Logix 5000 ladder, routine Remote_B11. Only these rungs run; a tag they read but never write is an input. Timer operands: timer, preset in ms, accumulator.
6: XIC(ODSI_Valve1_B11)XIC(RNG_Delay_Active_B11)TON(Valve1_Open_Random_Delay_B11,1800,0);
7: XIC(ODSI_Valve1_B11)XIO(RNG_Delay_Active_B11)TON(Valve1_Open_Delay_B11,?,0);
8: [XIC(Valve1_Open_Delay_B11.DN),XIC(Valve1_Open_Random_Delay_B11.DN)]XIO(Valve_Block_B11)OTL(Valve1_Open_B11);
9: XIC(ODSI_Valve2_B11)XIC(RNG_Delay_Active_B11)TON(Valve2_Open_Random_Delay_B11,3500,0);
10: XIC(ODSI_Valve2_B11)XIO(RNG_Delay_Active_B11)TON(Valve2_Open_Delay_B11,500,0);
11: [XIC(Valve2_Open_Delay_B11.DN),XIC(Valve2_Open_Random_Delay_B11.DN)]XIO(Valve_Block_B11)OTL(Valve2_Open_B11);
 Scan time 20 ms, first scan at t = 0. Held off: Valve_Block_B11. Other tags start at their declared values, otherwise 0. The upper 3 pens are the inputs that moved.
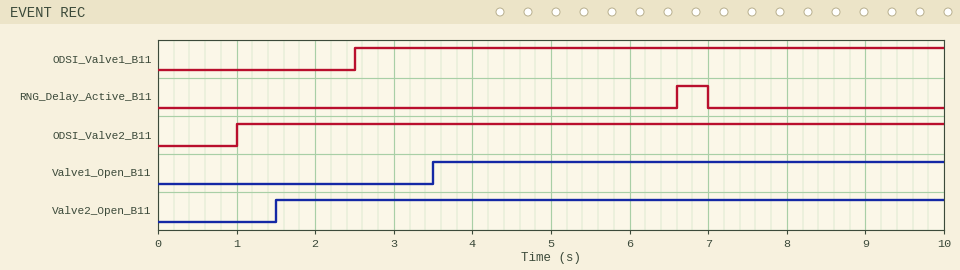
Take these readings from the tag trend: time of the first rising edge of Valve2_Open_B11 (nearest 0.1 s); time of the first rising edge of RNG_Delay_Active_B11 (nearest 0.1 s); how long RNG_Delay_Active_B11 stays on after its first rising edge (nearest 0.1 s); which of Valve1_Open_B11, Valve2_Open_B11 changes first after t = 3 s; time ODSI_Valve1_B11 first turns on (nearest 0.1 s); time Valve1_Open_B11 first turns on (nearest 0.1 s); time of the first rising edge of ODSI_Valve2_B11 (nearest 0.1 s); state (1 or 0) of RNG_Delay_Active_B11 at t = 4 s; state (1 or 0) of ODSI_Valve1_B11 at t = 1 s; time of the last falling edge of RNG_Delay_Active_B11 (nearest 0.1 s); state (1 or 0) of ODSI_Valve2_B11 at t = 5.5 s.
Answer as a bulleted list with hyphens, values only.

- 1.5 s
- 6.6 s
- 0.4 s
- Valve1_Open_B11
- 2.5 s
- 3.5 s
- 1.0 s
- 0
- 0
- 7.0 s
- 1
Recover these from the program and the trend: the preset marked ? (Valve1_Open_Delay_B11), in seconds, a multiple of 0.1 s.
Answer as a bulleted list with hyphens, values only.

- 1.0 s
